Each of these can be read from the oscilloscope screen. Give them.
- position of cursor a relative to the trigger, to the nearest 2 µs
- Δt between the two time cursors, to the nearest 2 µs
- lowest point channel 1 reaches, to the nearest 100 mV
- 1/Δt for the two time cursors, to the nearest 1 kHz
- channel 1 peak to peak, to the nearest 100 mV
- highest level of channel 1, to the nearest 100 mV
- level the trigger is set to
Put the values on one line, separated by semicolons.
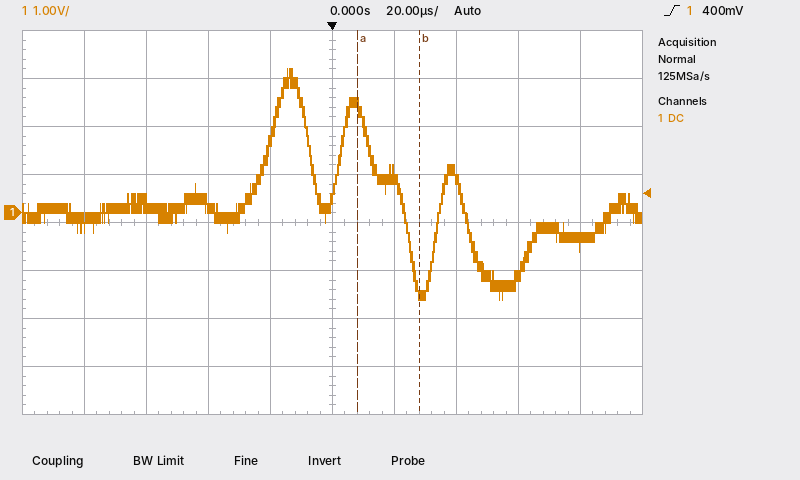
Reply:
+8 µs; 20 µs; -1.8 V; 50 kHz; 4.8 V; 3.0 V; 400 mV
